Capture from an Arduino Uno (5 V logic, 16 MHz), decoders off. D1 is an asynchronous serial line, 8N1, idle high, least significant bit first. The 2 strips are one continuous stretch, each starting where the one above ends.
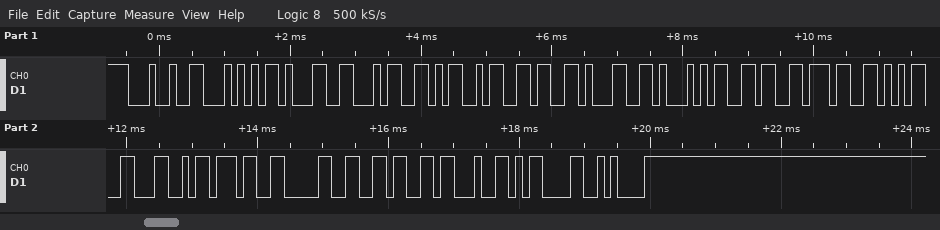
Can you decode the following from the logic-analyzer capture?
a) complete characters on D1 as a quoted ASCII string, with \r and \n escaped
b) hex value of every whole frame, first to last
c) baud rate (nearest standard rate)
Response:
"$T14M61Q675L706#\r\n"
0x24 0x54 0x31 0x34 0x4D 0x36 0x31 0x51 0x36 0x37 0x35 0x4C 0x37 0x30 0x36 0x23 0x0D 0x0A
9600 baud
